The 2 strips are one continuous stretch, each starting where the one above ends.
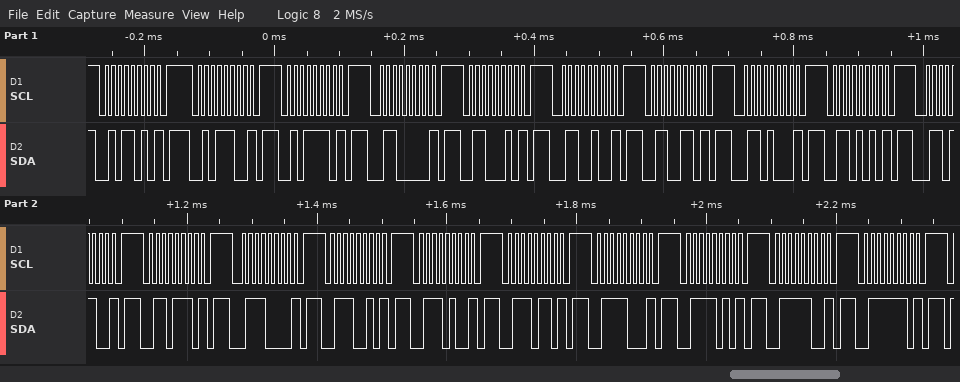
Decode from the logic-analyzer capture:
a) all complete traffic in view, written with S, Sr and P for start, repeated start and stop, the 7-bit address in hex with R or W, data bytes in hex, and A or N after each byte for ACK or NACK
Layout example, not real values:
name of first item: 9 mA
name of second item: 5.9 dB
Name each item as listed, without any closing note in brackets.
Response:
all complete traffic in view, written with S, Sr and P for start, repeated start and stop, the 7-bit address in hex with R or W, data bytes in hex, and A or N after each byte for ACK or NACK: S 2DW N P S 2EW N P S 2FW N P S 30W N P S 31W N P S 32W N P S 33W N P S 34W N P S 35W N P S 36W N P S 37W N P S 38W N P S 39W N P S 3AW N P S 3BW N P S 3CW N P S 3DW N P S 3EW N P S 3FW N P
